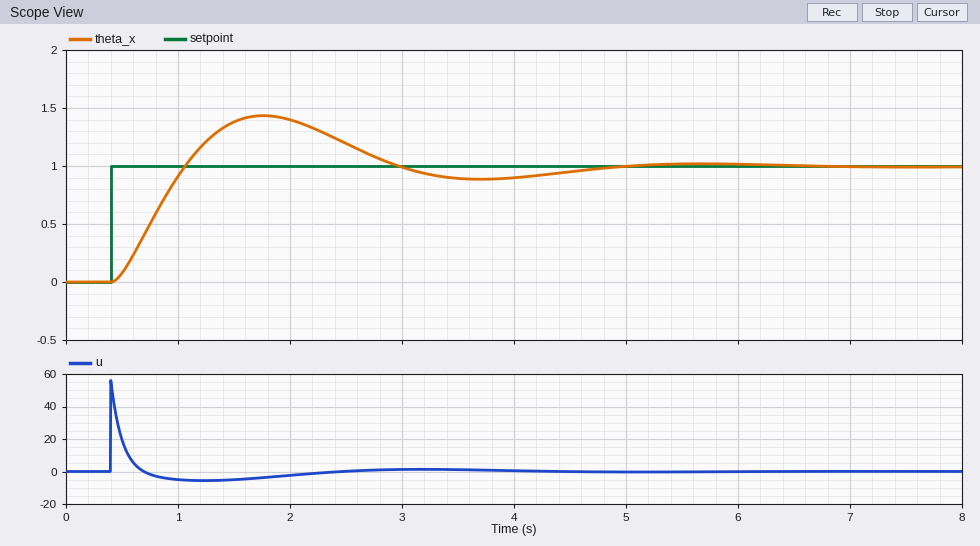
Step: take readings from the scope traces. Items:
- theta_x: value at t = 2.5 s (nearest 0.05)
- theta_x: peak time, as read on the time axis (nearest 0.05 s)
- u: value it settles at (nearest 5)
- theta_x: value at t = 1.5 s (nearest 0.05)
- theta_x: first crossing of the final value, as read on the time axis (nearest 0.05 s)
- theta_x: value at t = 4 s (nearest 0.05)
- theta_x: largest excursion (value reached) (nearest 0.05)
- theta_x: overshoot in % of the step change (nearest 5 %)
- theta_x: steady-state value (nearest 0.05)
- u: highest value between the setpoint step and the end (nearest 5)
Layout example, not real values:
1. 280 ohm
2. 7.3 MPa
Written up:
1. 1.20
2. 1.75 s
3. 0
4. 1.40
5. 1.05 s
6. 0.90
7. 1.45
8. 45 %
9. 1.00
10. 55
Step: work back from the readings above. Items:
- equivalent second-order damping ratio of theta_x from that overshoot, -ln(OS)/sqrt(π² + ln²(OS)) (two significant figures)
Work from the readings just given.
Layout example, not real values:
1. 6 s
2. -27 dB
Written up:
1. 0.25
